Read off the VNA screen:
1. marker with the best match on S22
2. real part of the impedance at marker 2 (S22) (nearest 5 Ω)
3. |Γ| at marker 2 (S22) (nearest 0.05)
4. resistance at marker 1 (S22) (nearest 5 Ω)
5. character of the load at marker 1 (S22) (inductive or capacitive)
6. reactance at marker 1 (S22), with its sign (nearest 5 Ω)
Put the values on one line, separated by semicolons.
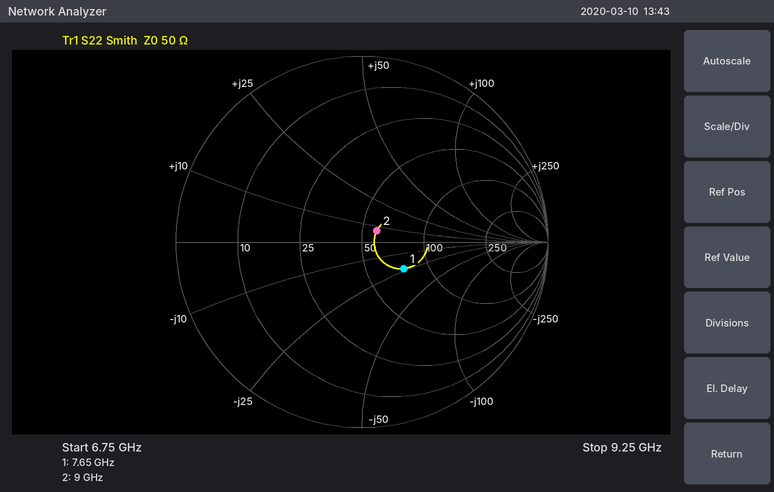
marker 2; 60 Ω; 0.10; 75 Ω; capacitive; -25 Ω
